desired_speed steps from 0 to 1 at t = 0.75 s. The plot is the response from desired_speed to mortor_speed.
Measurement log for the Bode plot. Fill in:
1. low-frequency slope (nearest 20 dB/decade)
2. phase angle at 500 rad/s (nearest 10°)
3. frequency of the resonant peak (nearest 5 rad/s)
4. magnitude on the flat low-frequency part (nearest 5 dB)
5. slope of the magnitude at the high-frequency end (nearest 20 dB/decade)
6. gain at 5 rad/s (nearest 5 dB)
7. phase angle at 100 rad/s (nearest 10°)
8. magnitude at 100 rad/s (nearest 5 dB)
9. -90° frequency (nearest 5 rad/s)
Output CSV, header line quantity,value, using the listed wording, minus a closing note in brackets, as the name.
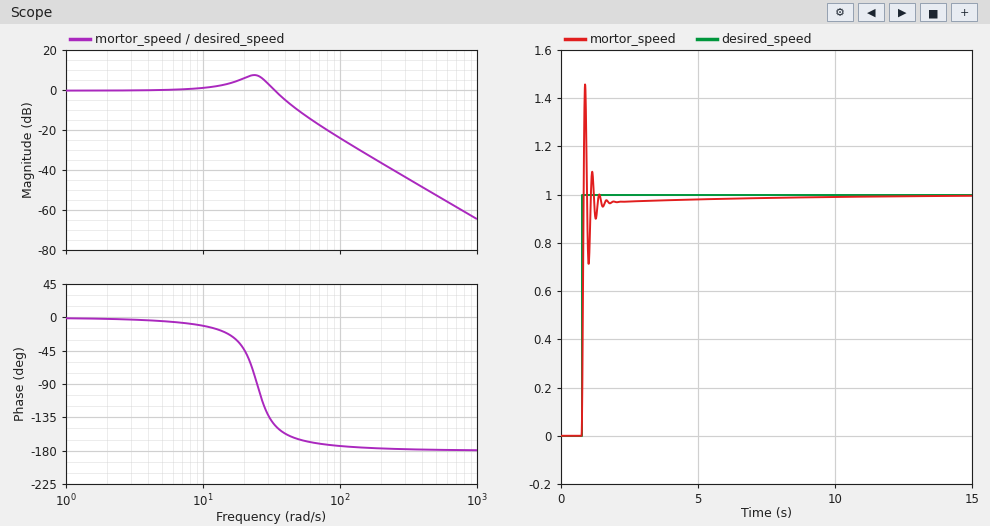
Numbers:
quantity,value
low-frequency slope,0 dB/decade
phase angle at 500 rad/s,-180°
frequency of the resonant peak,25 rad/s
magnitude on the flat low-frequency part,0 dB
slope of the magnitude at the high-frequency end,-40 dB/decade
gain at 5 rad/s,0 dB
phase angle at 100 rad/s,-170°
magnitude at 100 rad/s,-25 dB
-90° frequency,25 rad/s
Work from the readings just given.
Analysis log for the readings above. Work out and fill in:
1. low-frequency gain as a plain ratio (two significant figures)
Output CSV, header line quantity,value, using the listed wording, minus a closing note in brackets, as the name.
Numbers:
quantity,value
low-frequency gain as a plain ratio,1.0
